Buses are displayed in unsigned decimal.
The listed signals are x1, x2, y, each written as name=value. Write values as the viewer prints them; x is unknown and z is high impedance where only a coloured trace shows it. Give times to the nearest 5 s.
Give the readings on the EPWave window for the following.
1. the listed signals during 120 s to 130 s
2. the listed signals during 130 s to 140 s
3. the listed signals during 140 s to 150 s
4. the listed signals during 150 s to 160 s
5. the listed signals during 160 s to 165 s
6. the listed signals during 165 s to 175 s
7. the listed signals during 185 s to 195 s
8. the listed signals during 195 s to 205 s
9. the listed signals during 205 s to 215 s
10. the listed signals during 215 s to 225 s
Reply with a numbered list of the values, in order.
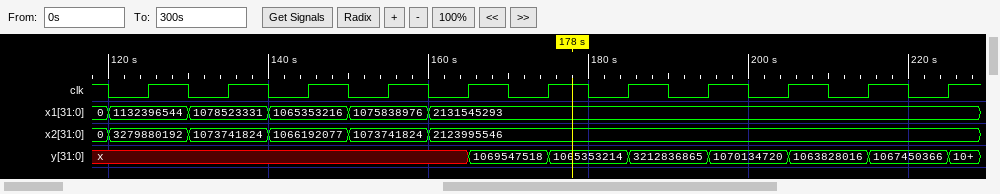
1. x1=1132396544, x2=3279880192, y=x
2. x1=1078523331, x2=1073741824, y=x
3. x1=1065353216, x2=1066192077, y=x
4. x1=1075838976, x2=1073741824, y=x
5. x1=2131545293, x2=2123995546, y=x
6. x1=2131545293, x2=2123995546, y=1069547518
7. x1=2131545293, x2=2123995546, y=3212836865
8. x1=2131545293, x2=2123995546, y=1070134720
9. x1=2131545293, x2=2123995546, y=1063828016
10. x1=2131545293, x2=2123995546, y=1067450366
